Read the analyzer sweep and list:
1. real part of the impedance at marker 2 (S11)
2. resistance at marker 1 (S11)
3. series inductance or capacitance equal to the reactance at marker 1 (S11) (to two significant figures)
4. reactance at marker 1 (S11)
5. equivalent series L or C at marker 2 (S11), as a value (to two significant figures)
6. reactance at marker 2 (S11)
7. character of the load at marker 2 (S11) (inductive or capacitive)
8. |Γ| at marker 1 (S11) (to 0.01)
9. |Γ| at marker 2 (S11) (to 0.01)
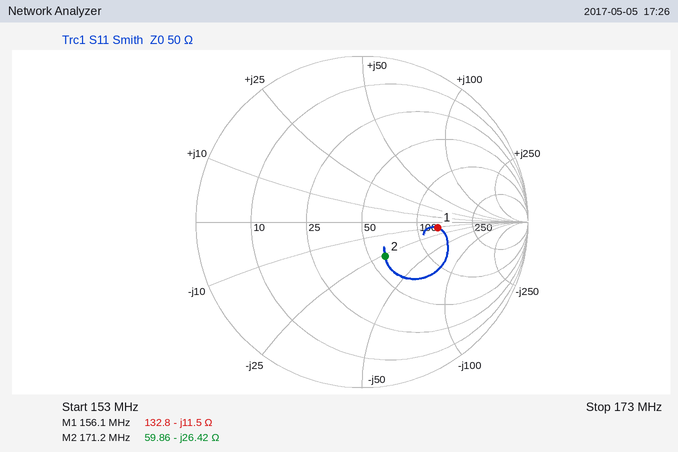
59.86 Ω
132.8 Ω
89 pF
-11.5 Ω
35 pF
-26.42 Ω
capacitive
0.46
0.25
